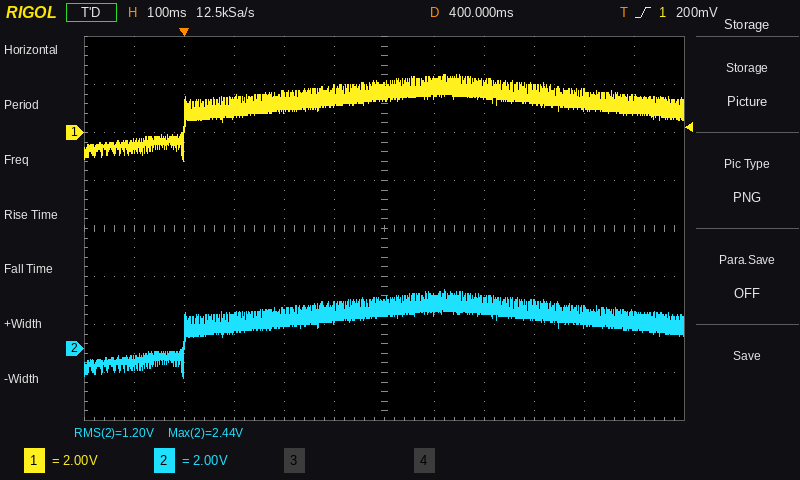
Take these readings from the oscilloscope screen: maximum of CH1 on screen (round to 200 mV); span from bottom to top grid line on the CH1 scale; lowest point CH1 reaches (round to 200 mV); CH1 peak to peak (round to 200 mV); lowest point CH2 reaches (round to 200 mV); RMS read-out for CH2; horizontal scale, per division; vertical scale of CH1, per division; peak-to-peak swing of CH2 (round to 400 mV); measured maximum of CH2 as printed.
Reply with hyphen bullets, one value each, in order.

- 2.4 V
- 16 V
- -1.2 V
- 3.6 V
- -1.2 V
- 1.20 V
- 100 ms
- 2 V
- 3.6 V
- 2.44 V
